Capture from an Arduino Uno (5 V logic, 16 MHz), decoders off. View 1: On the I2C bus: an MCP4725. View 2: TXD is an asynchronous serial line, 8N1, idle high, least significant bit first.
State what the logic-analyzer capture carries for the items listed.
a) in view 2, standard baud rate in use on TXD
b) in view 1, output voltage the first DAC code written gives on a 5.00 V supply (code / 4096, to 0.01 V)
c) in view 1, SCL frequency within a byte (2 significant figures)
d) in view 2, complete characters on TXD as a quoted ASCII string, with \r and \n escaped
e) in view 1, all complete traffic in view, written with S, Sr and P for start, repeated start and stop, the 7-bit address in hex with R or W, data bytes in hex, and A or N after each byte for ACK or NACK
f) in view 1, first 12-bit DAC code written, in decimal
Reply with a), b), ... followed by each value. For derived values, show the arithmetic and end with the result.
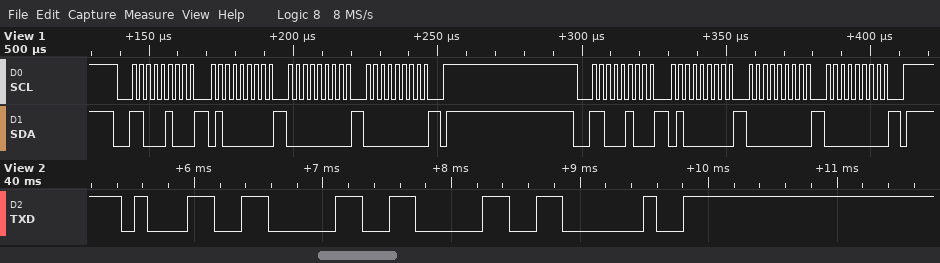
a) 9600 baud
b) 0 / 4096 x 5.00 V = 0.00 V
c) 400 kHz
d) "100 "
e) S 62W A 40 A 00 A 00 A P S 62W A 40 A 00 A 00 A P
f) 0
